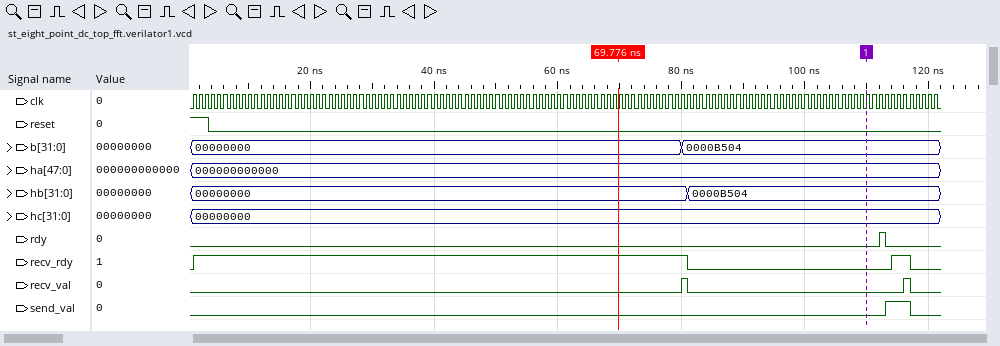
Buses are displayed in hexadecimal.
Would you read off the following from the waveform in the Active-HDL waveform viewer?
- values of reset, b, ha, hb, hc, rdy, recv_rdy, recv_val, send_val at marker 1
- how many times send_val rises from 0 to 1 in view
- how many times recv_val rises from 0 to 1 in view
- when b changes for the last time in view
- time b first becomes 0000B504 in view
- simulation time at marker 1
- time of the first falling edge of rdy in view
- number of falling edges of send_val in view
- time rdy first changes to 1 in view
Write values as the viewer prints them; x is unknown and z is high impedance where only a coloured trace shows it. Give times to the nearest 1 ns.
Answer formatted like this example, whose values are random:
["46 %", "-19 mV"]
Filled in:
["reset=0, b=0000B504, ha=000000000000, hb=0000B504, hc=00000000, rdy=0, recv_rdy=0, recv_val=0, send_val=0", "1", "2", "80 ns", "80 ns", "110 ns", "113 ns", "1", "112 ns"]
